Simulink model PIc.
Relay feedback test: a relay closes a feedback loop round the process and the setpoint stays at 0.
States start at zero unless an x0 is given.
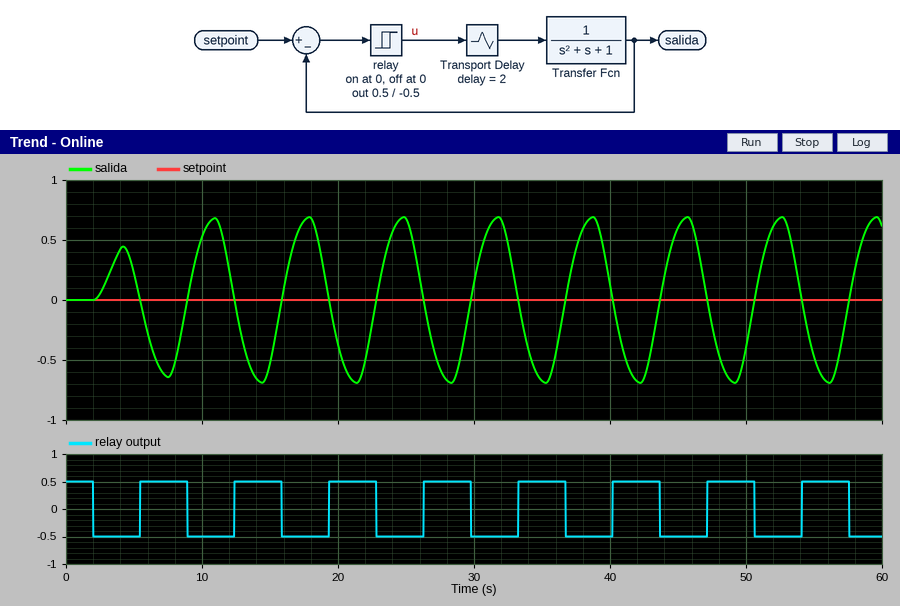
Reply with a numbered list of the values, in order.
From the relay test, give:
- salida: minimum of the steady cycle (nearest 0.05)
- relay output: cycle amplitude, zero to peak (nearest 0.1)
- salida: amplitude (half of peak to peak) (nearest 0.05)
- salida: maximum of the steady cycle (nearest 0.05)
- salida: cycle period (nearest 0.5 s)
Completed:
1. -0.70
2. 0.5
3. 0.70
4. 0.70
5. 7.0 s
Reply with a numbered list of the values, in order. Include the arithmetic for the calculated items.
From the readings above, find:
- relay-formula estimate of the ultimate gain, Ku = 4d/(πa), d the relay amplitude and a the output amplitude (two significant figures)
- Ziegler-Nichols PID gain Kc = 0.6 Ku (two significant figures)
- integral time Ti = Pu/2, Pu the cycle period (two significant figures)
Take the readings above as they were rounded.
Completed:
1. 4 × 0.5 / (π × 0.7) = 0.91
2. 0.6 × 0.91 = 0.55
3. 7 / 2 = 3.5 s
